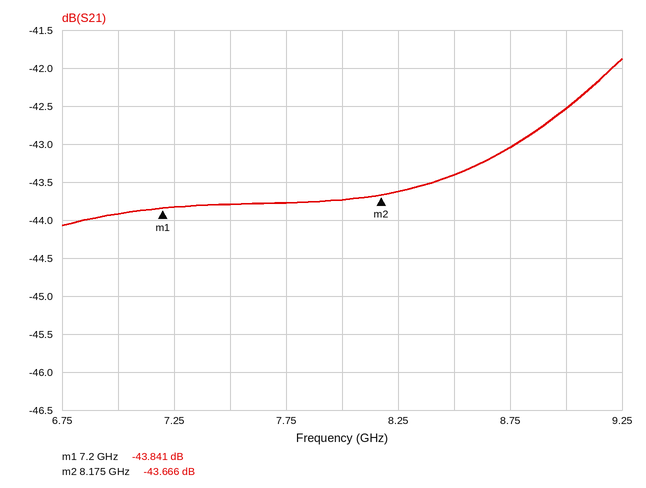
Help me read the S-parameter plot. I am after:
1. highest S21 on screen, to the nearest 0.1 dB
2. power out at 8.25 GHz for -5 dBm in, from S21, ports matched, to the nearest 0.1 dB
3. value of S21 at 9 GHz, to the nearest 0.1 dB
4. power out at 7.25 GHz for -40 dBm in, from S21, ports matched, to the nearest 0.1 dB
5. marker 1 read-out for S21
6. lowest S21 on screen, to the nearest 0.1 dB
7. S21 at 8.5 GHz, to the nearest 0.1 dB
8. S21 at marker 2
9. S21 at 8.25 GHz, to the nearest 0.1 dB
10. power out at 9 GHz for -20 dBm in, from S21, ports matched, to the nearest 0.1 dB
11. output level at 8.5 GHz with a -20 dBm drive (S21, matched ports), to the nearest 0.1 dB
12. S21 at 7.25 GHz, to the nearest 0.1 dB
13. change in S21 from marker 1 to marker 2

-41.9 dB
-48.6 dBm
-42.5 dB
-83.8 dBm
-43.841 dB
-44.1 dB
-43.4 dB
-43.666 dB
-43.6 dB
-62.5 dBm
-63.4 dBm
-43.8 dB
0.175 dB
